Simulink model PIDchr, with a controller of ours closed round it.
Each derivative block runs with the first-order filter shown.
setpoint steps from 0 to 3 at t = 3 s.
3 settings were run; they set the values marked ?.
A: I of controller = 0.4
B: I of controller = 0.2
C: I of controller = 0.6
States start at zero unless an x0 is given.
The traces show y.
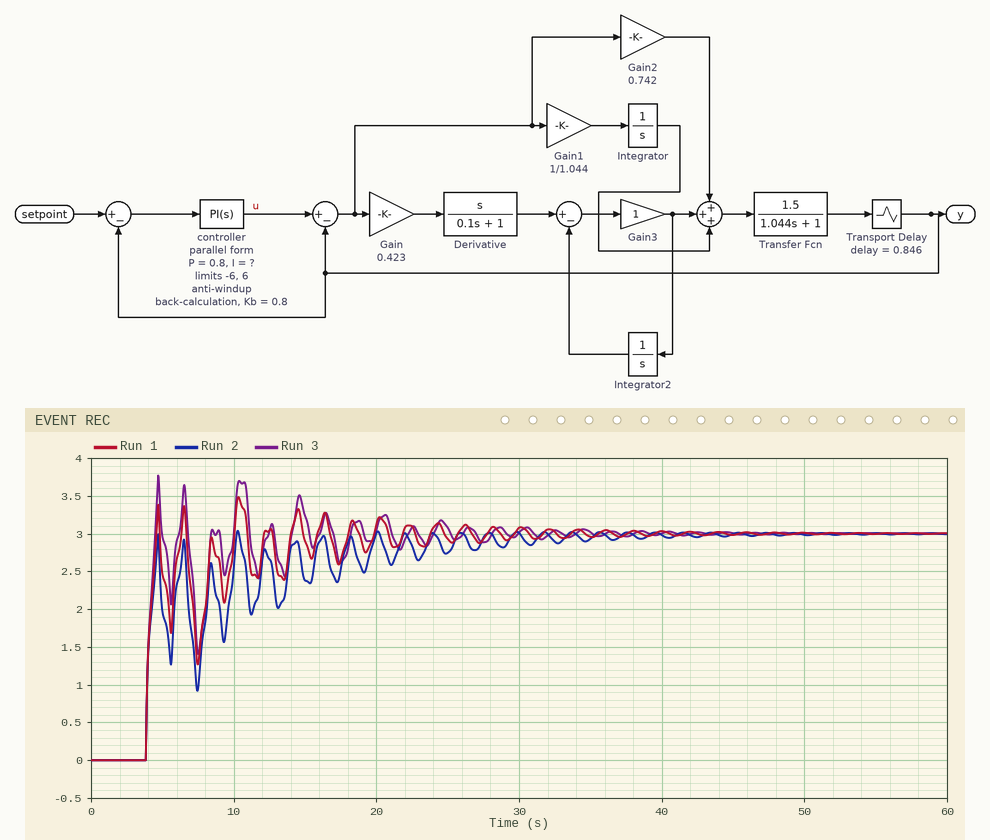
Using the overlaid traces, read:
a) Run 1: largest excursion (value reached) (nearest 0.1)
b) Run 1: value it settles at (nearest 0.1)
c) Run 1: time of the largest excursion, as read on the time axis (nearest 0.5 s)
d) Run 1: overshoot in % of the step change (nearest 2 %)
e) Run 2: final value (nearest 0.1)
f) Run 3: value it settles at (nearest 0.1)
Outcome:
3.5
3.0
10.5 s
16 %
3.0
3.0
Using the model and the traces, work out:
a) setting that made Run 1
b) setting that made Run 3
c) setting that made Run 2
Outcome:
A
C
B
